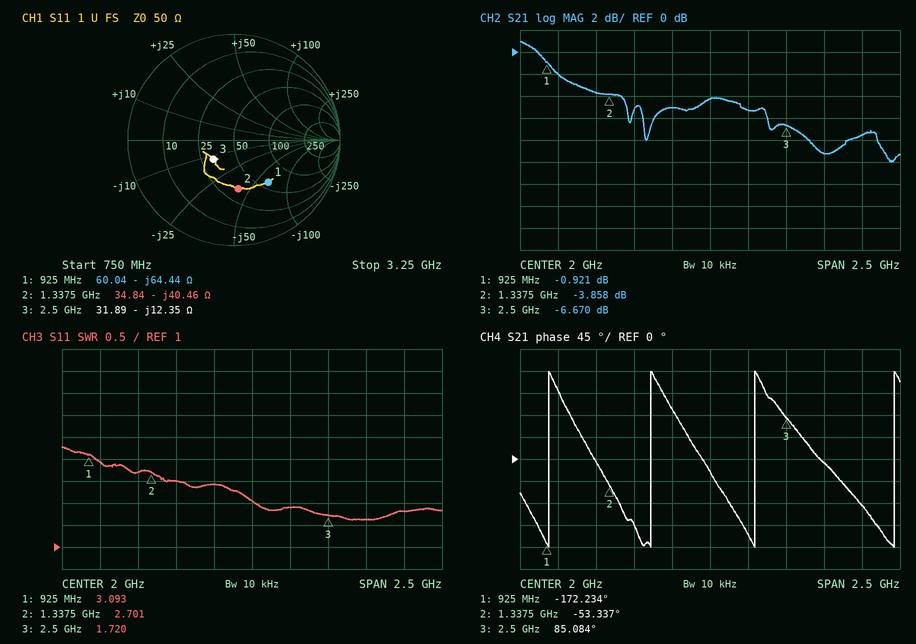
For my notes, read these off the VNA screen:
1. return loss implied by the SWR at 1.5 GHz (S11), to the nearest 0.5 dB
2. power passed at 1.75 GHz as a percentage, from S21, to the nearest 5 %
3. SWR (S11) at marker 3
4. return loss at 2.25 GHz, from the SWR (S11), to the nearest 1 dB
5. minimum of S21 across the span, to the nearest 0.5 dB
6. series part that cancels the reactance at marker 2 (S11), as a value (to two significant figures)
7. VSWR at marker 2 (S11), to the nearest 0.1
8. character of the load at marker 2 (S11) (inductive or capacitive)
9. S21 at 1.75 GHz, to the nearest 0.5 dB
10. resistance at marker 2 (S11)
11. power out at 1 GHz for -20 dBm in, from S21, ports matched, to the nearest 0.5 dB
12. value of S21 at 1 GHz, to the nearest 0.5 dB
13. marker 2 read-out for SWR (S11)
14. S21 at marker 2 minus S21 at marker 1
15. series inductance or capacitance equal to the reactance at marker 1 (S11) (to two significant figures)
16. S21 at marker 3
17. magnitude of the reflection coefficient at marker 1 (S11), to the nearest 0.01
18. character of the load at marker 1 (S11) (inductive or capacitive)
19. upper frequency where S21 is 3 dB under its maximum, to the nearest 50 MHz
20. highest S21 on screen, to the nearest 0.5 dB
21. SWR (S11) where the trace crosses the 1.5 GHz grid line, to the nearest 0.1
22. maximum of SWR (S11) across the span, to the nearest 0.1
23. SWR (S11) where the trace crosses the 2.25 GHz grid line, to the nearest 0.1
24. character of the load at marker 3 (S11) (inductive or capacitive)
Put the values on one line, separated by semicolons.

7.5 dB; 30 %; 1.720; 10 dB; -10.0 dB; 4.8 nH; 2.7; capacitive; -5.0 dB; 34.84 Ω; -22.0 dBm; -2.0 dB; 2.701; -2.937 dB; 2.7 pF; -6.670 dB; 0.51; capacitive; 1.00 GHz; 1.0 dB; 2.5; 3.3; 1.9; capacitive
